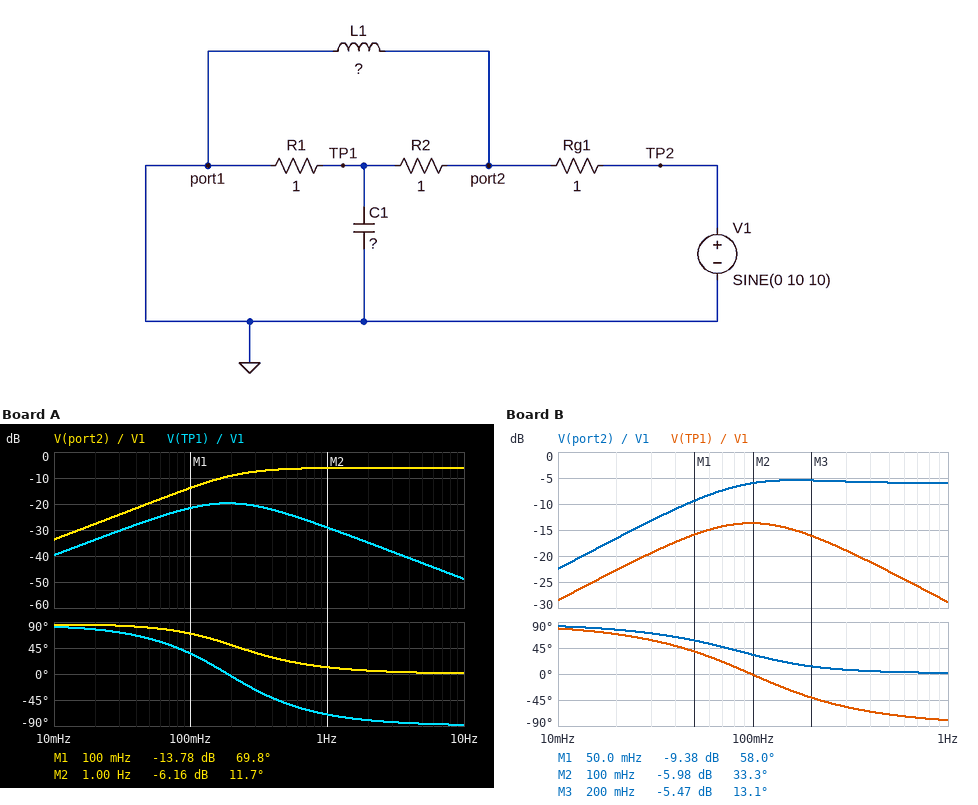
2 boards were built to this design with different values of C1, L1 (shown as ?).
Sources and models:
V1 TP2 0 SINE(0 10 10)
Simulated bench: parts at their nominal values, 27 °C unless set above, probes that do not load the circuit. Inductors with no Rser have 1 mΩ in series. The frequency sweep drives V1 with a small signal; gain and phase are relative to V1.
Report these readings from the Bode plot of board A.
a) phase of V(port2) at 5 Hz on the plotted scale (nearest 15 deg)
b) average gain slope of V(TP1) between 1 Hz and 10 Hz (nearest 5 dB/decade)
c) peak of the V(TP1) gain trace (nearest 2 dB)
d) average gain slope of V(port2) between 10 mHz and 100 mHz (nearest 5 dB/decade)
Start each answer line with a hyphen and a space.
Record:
- 0 deg
- -20 dB/decade
- -20 dB
- 20 dB/decade
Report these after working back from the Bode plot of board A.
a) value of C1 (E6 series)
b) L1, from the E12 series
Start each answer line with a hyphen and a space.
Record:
- 2.2 F
- 330 mH
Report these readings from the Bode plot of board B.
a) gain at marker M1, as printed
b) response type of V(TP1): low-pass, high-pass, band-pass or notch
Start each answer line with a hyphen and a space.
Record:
- -9.38 dB
- band-pass
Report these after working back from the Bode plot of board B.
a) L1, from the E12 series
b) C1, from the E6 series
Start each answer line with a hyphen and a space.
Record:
- 1.2 H
- 2.2 F
